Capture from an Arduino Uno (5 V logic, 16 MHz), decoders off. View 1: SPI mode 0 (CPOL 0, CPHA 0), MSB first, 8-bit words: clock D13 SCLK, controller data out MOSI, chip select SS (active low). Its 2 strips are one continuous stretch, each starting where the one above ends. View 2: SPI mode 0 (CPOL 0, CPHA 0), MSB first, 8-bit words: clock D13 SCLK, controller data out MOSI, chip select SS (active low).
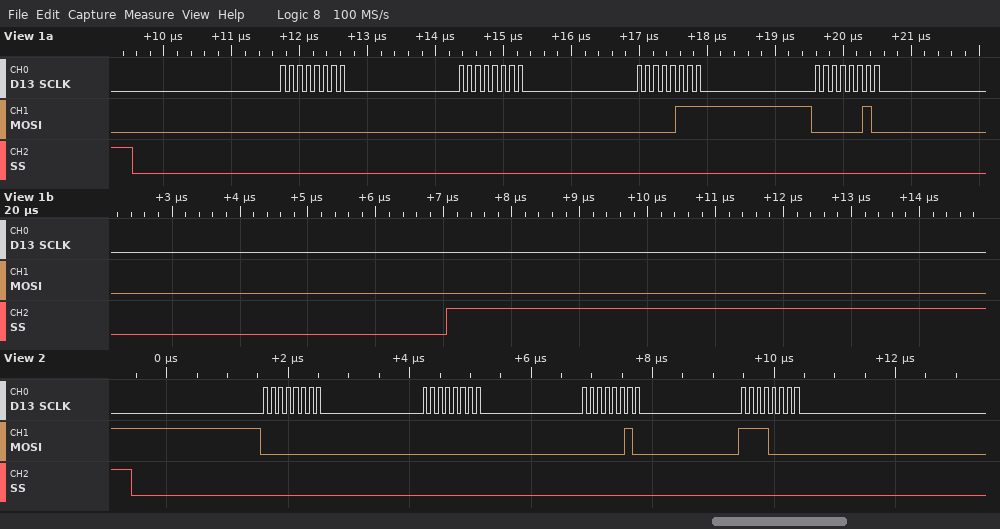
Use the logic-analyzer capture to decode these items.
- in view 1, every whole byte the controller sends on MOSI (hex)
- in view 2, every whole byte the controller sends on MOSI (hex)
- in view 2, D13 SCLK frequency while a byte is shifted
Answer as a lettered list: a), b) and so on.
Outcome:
a) 0x00 0x00 0x07 0x02
b) 0x00 0x00 0x02 0xF0
c) 8 MHz
